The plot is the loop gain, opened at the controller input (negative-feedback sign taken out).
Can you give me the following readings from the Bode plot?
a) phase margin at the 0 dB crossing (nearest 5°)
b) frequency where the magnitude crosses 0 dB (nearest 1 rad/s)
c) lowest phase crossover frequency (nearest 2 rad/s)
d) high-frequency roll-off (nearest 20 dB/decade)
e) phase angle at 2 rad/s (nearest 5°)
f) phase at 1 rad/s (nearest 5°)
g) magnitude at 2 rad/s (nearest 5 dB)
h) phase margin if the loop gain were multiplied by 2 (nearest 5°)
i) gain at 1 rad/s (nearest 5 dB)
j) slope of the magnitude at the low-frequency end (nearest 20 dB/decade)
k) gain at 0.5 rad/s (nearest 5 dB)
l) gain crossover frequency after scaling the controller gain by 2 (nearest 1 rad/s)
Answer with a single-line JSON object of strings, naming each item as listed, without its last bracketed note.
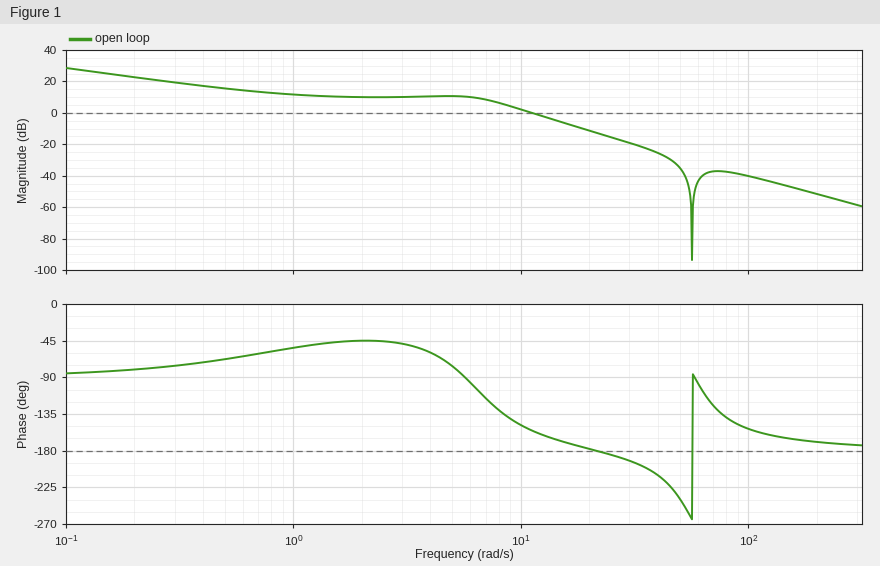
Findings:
{"phase margin at the 0 dB crossing": "25°", "frequency where the magnitude crosses 0 dB": "11 rad/s", "lowest phase crossover frequency": "22 rad/s", "high-frequency roll-off": "-40 dB/decade", "phase angle at 2 rad/s": "-45°", "phase at 1 rad/s": "-55°", "magnitude at 2 rad/s": "10 dB", "phase margin if the loop gain were multiplied by 2": "10°", "gain at 1 rad/s": "10 dB", "slope of the magnitude at the low-frequency end": "-20 dB/decade", "gain at 0.5 rad/s": "15 dB", "gain crossover frequency after scaling the controller gain by 2": "15 rad/s"}
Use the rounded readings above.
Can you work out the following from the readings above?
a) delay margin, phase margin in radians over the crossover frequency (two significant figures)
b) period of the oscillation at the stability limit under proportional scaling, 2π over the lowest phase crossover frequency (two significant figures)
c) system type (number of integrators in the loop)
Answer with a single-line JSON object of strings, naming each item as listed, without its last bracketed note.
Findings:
{"delay margin, phase margin in radians over the crossover frequency": "0.040 s", "period of the oscillation at the stability limit under proportional scaling, 2π over the lowest phase crossover frequency": "0.29 s", "system type": "1"}
